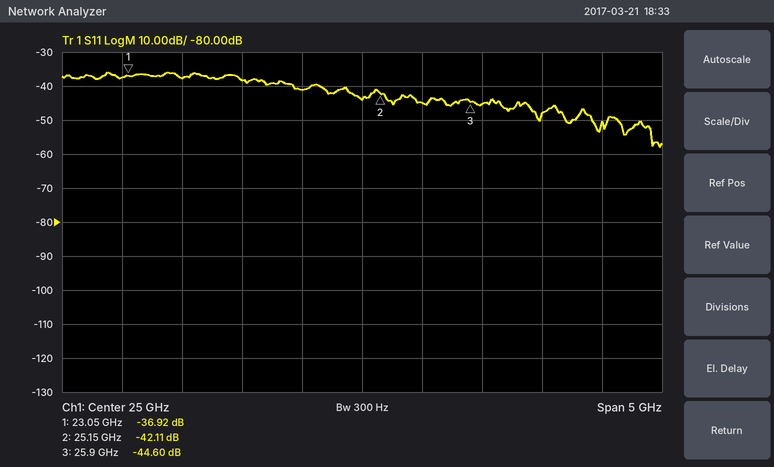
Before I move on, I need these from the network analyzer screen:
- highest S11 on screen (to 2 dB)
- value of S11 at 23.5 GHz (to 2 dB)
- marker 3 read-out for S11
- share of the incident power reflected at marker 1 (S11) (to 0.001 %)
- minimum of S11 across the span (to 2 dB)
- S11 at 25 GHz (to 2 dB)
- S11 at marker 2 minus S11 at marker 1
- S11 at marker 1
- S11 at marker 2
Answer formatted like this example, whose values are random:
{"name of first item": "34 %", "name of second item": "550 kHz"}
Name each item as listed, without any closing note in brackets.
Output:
{"highest S11 on screen": "-36 dB", "value of S11 at 23.5 GHz": "-38 dB", "marker 3 read-out for S11": "-44.60 dB", "share of the incident power reflected at marker 1 (S11)": "0.020 %", "minimum of S11 across the span": "-58 dB", "S11 at 25 GHz": "-44 dB", "S11 at marker 2 minus S11 at marker 1": "-5.19 dB", "S11 at marker 1": "-36.92 dB", "S11 at marker 2": "-42.11 dB"}
